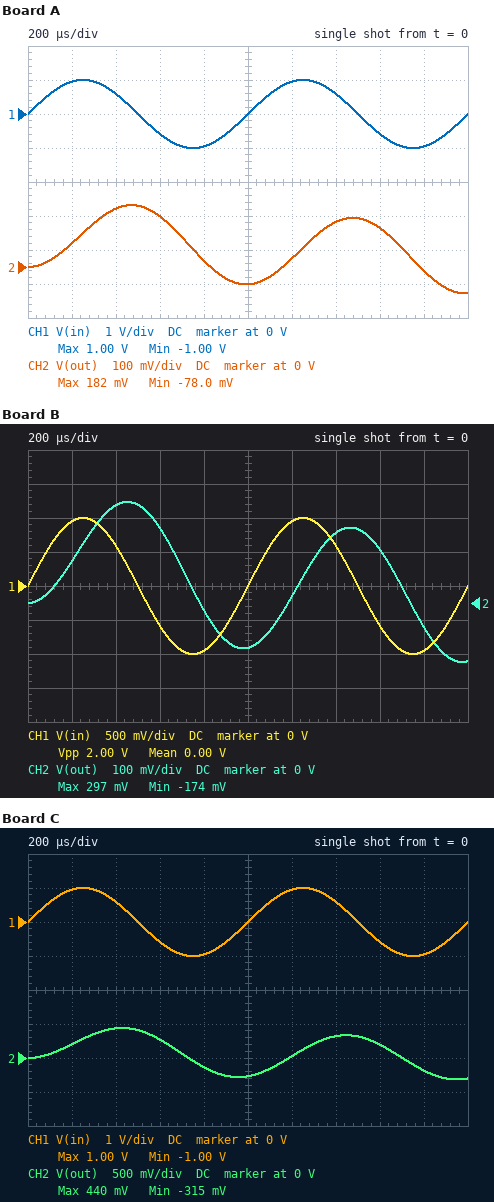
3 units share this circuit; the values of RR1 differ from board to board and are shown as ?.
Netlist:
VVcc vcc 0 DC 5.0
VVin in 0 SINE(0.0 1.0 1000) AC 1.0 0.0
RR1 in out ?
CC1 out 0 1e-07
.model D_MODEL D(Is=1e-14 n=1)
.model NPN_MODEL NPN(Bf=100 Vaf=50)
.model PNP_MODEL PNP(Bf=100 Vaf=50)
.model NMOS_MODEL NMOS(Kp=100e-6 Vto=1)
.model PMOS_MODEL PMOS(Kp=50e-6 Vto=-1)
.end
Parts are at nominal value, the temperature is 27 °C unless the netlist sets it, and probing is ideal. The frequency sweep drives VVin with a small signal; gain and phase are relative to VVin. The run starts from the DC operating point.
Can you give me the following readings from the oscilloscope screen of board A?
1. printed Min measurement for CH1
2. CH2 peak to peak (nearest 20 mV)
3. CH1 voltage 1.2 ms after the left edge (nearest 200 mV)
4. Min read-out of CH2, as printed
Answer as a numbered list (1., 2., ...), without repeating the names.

1. -1.00 V
2. 260 mV
3. 1.0 V
4. -78.0 mV
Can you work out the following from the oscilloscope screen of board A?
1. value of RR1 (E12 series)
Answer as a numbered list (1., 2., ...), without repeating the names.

1. 15 kΩ
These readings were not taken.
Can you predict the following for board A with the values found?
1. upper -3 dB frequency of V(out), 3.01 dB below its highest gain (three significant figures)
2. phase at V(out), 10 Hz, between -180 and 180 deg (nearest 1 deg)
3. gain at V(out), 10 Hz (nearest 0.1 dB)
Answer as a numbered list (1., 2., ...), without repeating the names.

1. 106 Hz
2. -5 deg
3. 0 dB
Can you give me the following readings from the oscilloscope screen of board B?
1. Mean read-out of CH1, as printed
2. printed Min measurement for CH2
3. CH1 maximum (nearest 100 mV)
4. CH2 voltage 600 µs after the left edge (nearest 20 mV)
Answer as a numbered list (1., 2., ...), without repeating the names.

1. 0.00 V
2. -174 mV
3. 1.0 V
4. 220 mV
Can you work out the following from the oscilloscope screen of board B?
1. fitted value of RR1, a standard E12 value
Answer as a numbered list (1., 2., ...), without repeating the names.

1. 8.2 kΩ
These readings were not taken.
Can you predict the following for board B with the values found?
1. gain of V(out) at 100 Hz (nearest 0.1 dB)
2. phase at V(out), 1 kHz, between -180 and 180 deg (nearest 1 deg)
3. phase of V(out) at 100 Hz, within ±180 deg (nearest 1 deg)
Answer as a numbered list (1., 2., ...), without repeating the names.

1. -1.0 dB
2. -79 deg
3. -27 deg
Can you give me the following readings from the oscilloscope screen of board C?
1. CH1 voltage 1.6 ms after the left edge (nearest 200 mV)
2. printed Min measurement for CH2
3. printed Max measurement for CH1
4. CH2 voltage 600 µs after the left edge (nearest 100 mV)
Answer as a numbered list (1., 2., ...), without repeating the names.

1. -600 mV
2. -315 mV
3. 1.00 V
4. 300 mV
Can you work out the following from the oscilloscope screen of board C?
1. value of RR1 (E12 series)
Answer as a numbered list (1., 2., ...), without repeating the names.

1. 4.7 kΩ
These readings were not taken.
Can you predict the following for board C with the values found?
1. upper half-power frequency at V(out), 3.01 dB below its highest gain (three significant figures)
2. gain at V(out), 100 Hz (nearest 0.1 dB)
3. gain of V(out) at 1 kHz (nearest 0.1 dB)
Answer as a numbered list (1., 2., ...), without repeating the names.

1. 339 Hz
2. -0.4 dB
3. -9.9 dB
